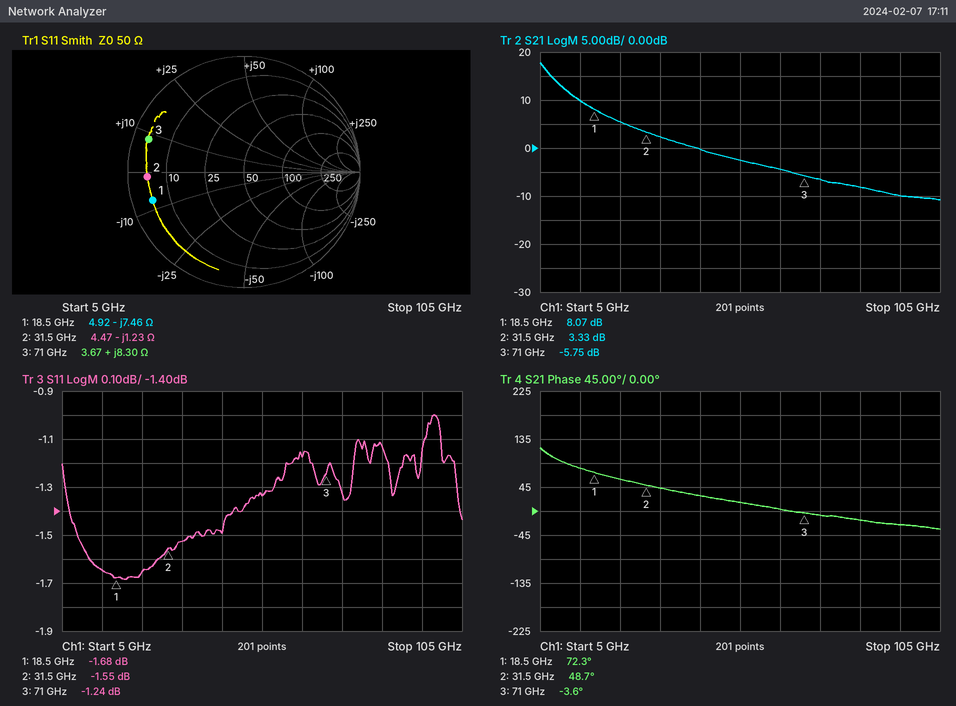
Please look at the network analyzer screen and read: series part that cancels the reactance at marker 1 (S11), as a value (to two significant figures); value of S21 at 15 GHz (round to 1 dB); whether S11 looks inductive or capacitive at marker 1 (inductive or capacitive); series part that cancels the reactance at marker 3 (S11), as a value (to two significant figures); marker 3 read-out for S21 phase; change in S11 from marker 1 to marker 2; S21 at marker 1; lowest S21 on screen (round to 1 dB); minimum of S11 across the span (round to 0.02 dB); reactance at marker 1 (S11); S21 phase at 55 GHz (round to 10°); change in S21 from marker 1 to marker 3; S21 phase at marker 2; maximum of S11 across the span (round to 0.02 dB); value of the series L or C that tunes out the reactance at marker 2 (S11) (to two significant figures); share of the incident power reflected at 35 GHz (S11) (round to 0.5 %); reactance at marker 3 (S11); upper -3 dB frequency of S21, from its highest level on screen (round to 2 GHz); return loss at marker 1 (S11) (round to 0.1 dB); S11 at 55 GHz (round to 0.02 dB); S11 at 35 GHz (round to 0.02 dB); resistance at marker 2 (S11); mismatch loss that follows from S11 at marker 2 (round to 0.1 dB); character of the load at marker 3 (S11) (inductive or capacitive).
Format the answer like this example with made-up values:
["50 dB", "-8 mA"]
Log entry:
["64 pH", "10 dB", "capacitive", "270 fF", "-3.6°", "0.13 dB", "8.07 dB", "-11 dB", "-1.68 dB", "-7.46 Ω", "20°", "-13.82 dB", "48.7°", "-1.00 dB", "6.2 pH", "70.5 %", "+8.30 Ω", "8 GHz", "1.7 dB", "-1.34 dB", "-1.52 dB", "4.47 Ω", "5.2 dB", "inductive"]
